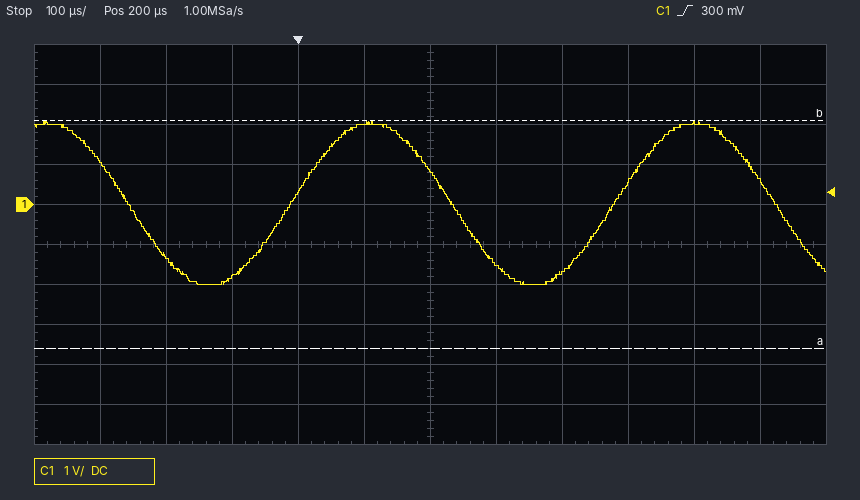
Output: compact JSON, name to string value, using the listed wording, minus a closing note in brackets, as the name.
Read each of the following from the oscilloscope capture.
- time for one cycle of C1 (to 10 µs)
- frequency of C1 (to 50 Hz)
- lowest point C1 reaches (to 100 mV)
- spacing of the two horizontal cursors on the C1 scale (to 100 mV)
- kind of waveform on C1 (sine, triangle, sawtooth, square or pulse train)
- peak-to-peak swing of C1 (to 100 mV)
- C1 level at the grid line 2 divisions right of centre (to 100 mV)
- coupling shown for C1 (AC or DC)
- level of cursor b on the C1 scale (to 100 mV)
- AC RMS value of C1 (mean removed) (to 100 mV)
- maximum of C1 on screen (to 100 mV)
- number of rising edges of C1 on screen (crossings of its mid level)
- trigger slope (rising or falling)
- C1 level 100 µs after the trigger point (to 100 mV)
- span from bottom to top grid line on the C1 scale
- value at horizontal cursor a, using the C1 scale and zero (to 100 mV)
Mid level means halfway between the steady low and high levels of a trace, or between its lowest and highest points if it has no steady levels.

{"time for one cycle of C1": "490 µs", "frequency of C1": "2.05 kHz", "lowest point C1 reaches": "-2.0 V", "spacing of the two horizontal cursors on the C1 scale": "5.7 V", "kind of waveform on C1": "sine", "peak-to-peak swing of C1": "4.1 V", "C1 level at the grid line 2 divisions right of centre": "-1.7 V", "coupling shown for C1": "DC", "level of cursor b on the C1 scale": "2.1 V", "AC RMS value of C1 (mean removed)": "1.4 V", "maximum of C1 on screen": "2.1 V", "number of rising edges of C1 on screen": "2", "trigger slope": "rising", "C1 level 100 µs after the trigger point": "2.0 V", "span from bottom to top grid line on the C1 scale": "10 V", "value at horizontal cursor a, using the C1 scale and zero": "-3.6 V"}
